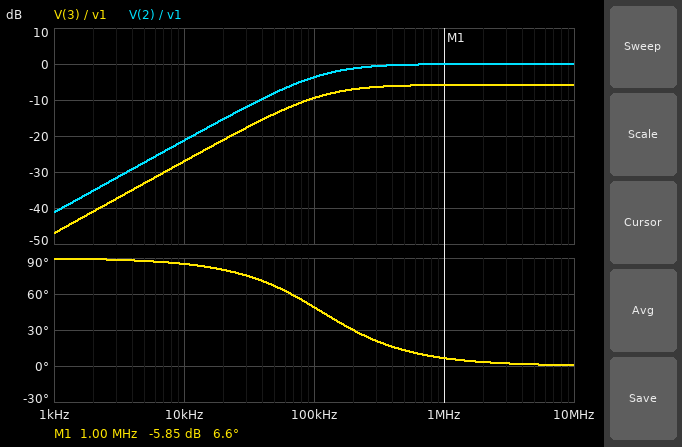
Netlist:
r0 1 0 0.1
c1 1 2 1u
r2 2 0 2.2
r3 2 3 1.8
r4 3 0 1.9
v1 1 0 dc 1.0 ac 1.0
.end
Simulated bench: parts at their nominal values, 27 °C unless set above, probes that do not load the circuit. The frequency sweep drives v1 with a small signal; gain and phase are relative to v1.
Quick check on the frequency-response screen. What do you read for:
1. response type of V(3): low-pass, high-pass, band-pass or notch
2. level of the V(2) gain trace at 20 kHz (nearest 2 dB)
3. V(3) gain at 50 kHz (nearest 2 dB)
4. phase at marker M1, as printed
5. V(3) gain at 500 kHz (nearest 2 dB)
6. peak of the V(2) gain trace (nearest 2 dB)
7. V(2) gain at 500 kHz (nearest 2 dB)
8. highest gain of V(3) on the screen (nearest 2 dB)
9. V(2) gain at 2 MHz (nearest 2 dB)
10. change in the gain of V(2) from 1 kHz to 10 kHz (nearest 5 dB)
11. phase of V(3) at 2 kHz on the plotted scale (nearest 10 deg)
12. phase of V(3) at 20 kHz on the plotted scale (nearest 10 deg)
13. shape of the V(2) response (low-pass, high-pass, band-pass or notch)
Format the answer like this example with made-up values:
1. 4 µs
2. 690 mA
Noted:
1. high-pass
2. -16 dB
3. -14 dB
4. 6.6 deg
5. -6 dB
6. 0 dB
7. 0 dB
8. -6 dB
9. 0 dB
10. 20 dB
11. 90 deg
12. 80 deg
13. high-pass
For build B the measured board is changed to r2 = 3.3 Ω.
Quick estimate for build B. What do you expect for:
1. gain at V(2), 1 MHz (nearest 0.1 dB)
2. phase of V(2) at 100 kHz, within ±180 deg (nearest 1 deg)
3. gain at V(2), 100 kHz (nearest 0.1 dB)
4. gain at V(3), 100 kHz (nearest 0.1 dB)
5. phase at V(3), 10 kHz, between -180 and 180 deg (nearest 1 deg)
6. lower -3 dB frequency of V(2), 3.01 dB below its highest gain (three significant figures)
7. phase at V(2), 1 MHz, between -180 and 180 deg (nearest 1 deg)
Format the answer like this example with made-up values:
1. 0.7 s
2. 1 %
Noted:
1. 0 dB
2. 42 deg
3. -2.6 dB
4. -8.4 dB
5. 84 deg
6. 91.2 kHz
7. 5 deg
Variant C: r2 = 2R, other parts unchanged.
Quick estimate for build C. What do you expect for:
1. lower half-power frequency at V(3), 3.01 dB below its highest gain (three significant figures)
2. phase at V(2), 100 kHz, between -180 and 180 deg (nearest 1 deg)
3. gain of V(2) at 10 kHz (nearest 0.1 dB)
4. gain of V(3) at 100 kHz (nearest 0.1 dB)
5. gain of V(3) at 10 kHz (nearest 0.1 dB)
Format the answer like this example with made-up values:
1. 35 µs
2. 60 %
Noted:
1. 123 kHz
2. 51 deg
3. -21.8 dB
4. -9.8 dB
5. -27.6 dB
